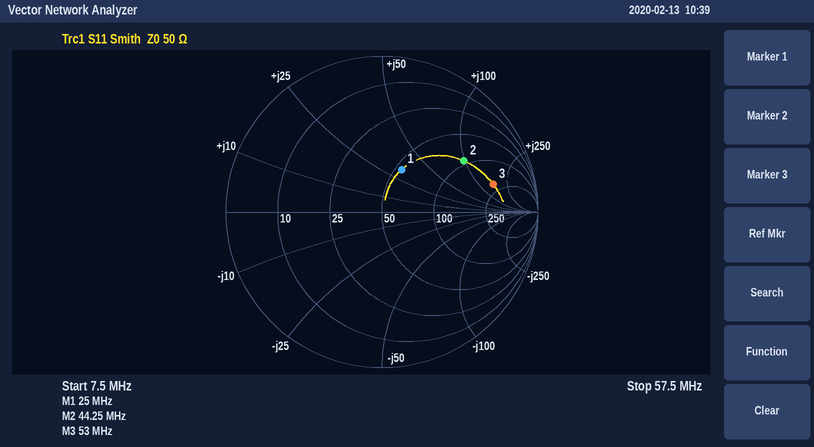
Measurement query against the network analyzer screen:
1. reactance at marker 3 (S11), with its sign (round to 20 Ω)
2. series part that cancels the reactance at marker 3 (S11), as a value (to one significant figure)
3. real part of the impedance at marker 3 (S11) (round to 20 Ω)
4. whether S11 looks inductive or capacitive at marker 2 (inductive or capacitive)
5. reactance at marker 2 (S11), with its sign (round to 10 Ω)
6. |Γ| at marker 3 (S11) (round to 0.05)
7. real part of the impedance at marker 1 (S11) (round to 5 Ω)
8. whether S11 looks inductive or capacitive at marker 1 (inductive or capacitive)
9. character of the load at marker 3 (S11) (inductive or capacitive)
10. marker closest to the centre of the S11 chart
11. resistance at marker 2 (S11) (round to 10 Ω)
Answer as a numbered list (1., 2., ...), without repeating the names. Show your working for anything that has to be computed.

1. +160 Ω
2. C = 1/(2π × 53 MHz × 160 Ω) ≈ 18.8 pF, so 20 pF to one significant figure
3. 200 Ω
4. inductive
5. +100 Ω
6. 0.75
7. 55 Ω
8. inductive
9. inductive
10. marker 1
11. 90 Ω
